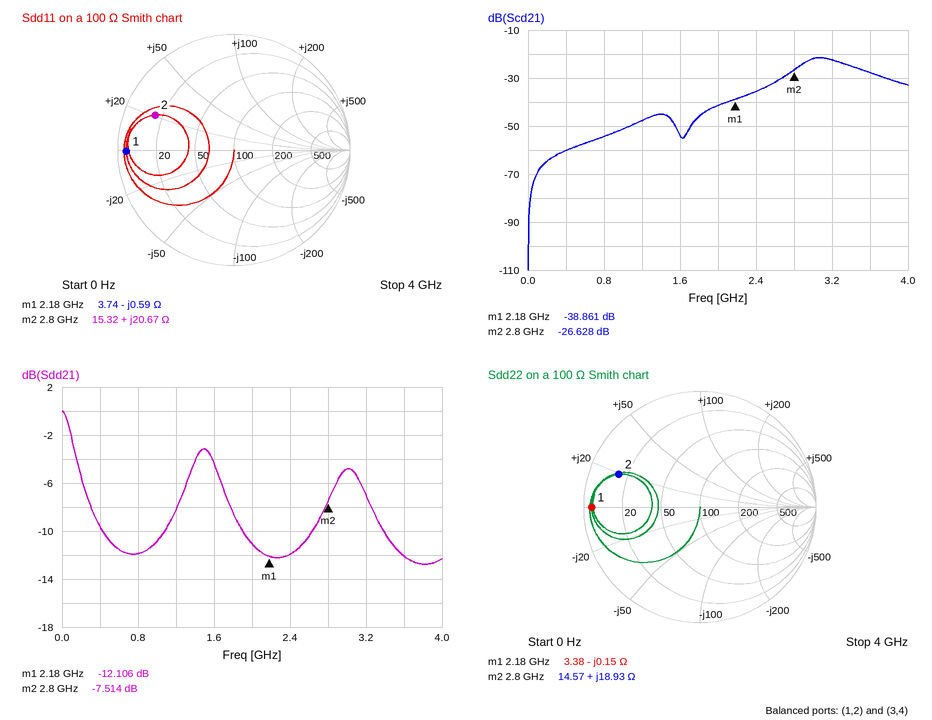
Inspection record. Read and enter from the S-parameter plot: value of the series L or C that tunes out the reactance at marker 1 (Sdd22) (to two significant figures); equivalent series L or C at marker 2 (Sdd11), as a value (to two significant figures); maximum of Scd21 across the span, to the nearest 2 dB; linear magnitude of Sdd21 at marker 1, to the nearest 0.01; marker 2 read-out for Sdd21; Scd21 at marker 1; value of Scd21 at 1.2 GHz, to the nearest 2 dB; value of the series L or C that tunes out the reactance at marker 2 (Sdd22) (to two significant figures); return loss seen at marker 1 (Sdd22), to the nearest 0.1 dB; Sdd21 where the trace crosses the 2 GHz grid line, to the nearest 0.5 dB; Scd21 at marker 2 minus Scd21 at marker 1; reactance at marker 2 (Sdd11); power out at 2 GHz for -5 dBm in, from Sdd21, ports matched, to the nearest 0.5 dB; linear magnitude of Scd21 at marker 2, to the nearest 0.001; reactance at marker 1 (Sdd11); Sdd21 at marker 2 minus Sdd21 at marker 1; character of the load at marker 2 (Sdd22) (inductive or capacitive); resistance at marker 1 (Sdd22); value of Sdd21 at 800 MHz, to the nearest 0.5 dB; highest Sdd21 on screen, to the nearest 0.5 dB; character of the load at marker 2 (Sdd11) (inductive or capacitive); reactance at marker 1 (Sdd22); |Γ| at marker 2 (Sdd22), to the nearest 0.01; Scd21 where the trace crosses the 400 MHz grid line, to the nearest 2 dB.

11 pH
1.2 nH
-22 dB
0.25
-7.514 dB
-38.861 dB
-48 dB
3.0 pF
0.6 dB
-11.0 dB
12.233 dB
+20.67 Ω
-16.0 dBm
0.047
-0.59 Ω
4.592 dB
inductive
3.38 Ω
-12.0 dB
0.0 dB
inductive
-0.15 Ω
0.75
-60 dB
